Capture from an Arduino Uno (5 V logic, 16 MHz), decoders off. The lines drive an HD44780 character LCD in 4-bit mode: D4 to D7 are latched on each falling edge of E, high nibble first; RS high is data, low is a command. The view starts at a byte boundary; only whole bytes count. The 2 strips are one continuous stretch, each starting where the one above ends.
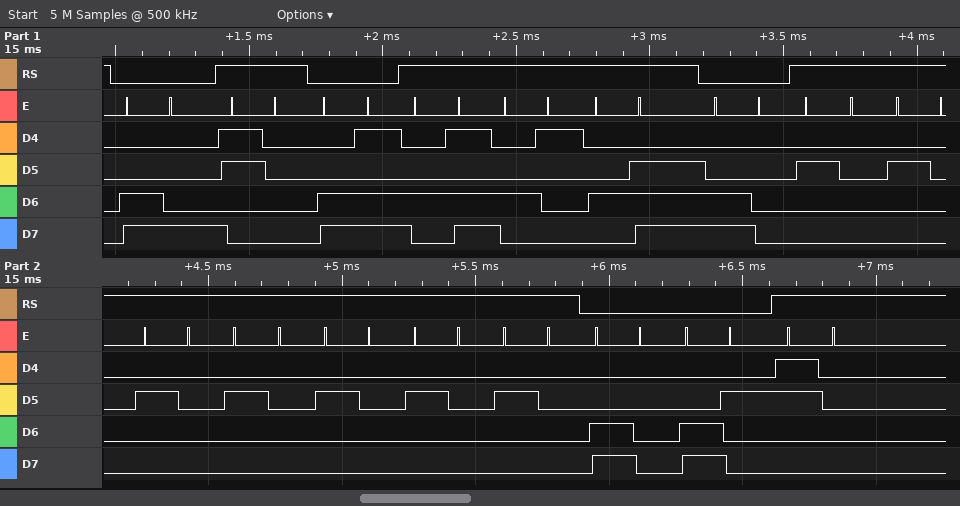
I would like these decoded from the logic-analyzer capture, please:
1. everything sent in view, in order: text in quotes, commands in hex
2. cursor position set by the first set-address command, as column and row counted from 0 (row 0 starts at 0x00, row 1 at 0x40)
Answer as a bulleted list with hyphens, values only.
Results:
- 0xC8 "0" 0xCD "MAN" 0xC0 "       " 0xC0 0xC2 "0"
- column 8, row 1
